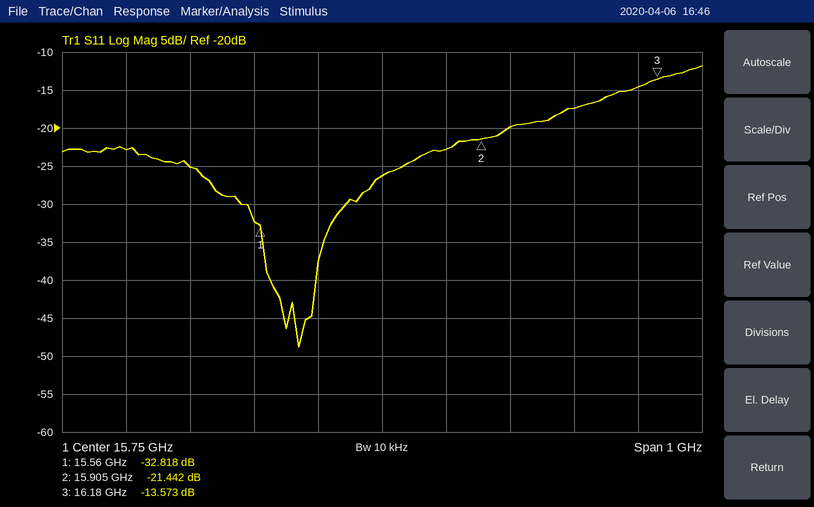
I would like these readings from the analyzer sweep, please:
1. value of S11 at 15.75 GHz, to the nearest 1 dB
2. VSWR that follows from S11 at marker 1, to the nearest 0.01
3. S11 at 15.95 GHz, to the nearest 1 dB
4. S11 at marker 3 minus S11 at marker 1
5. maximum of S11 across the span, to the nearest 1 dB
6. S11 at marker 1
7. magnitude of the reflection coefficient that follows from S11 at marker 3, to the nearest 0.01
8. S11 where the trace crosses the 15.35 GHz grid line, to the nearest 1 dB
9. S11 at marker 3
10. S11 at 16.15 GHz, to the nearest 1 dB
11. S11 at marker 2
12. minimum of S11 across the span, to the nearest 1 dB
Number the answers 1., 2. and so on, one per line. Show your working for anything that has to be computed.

1. -26 dB
2. (1 + 0.0229)/(1 − 0.0229) ≈ 1.05
3. -20 dB
4. -13.573 − (-32.818) = 19.245 dB
5. -12 dB
6. -32.818 dB
7. 10^(-13.573/20) ≈ 0.21
8. -23 dB
9. -13.573 dB
10. -15 dB
11. -21.442 dB
12. -49 dB
